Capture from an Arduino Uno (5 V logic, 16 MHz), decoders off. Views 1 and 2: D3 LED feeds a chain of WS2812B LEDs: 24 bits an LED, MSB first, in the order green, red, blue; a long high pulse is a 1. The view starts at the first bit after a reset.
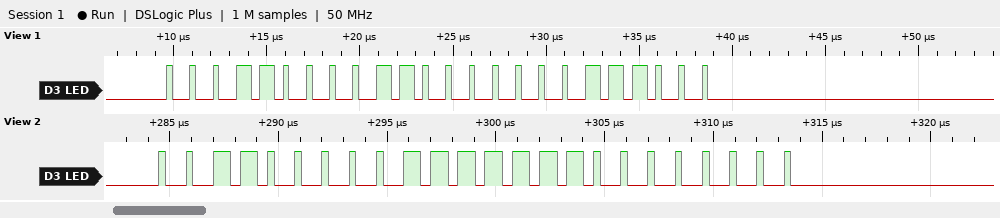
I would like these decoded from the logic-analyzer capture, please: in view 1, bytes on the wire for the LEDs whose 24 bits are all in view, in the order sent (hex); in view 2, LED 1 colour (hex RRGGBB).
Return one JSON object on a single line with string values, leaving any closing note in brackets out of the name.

{"in view 1, bytes on the wire for the LEDs whose 24 bits are all in view, in the order sent": "18 60 38", "in view 2, LED 1 colour": "#7F3000"}
